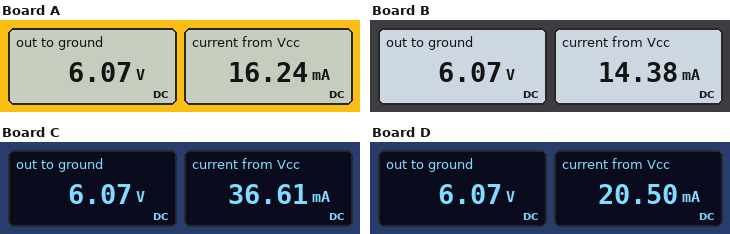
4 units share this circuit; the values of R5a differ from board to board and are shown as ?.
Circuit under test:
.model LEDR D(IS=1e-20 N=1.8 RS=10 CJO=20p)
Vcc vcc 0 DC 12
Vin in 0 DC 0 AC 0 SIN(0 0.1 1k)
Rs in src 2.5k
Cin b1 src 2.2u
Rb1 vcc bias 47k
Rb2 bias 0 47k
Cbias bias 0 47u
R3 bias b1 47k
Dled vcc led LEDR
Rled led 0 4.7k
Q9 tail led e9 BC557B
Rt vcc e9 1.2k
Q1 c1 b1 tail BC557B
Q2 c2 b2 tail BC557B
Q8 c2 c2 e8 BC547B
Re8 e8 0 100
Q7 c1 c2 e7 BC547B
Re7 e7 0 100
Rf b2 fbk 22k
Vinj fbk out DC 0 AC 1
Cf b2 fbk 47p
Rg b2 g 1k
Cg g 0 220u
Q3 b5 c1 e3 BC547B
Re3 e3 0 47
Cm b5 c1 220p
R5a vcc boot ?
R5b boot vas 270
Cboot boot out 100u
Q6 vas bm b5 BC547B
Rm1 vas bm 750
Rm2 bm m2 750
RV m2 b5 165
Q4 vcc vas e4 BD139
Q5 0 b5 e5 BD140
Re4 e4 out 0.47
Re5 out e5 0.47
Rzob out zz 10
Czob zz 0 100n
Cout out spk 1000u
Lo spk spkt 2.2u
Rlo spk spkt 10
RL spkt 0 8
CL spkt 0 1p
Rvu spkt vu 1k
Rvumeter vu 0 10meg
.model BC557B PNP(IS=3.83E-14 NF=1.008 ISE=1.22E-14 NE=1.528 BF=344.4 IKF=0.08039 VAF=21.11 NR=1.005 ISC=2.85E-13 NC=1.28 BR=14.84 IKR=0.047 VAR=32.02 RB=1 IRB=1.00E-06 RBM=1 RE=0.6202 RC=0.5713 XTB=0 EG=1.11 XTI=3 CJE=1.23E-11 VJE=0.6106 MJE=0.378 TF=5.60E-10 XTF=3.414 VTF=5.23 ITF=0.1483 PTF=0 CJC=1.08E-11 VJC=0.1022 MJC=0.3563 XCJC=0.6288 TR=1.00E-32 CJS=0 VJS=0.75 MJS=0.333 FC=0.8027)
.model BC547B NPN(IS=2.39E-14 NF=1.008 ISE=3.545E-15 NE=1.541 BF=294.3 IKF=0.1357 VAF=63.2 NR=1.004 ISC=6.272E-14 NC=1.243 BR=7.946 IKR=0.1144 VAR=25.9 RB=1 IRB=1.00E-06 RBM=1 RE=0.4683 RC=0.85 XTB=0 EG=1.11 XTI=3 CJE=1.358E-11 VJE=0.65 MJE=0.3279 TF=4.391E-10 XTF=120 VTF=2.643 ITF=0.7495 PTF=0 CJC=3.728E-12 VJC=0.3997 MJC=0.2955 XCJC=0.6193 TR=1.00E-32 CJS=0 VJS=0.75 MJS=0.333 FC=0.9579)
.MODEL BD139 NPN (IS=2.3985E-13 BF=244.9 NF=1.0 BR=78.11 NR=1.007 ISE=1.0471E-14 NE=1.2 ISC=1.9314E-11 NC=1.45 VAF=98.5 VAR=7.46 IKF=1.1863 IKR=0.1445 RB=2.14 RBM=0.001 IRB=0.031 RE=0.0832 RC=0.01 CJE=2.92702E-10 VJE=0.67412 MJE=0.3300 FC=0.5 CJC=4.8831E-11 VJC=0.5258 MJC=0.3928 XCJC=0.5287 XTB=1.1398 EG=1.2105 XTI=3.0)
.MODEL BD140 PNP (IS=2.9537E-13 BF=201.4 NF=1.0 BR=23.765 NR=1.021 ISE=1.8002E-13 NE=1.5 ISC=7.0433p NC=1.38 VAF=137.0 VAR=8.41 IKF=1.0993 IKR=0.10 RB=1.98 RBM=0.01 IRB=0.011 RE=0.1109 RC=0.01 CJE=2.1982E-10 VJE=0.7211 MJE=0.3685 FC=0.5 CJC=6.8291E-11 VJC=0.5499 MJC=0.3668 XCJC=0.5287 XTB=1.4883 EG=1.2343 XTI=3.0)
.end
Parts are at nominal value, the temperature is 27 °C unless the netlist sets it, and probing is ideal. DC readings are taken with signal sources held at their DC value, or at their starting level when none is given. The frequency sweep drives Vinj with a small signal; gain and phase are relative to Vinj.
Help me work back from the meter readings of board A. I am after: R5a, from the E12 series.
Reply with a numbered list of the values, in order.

1. 680 Ω
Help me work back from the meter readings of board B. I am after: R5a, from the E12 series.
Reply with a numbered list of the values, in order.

1. 820 Ω
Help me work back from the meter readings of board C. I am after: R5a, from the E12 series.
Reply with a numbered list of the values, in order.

1. 150 Ω
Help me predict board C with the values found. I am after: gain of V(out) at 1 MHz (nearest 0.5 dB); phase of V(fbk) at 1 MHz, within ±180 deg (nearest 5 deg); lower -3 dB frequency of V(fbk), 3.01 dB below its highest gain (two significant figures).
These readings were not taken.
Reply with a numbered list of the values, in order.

1. -2.0 dB
2. 40 deg
3. 4.2 MHz
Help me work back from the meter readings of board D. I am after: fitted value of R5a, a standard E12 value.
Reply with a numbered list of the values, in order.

1. 470 Ω
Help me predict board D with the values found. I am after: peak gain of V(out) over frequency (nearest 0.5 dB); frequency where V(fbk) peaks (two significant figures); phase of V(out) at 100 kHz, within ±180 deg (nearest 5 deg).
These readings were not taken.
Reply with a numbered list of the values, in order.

1. 0.5 dB
2. 5.5 MHz
3. 170 deg
